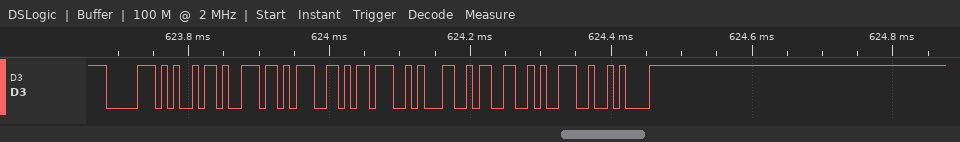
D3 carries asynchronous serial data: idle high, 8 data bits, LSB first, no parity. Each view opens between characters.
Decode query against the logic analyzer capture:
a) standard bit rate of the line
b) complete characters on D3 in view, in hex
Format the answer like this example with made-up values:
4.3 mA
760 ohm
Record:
115200 baud
70, 69, 6E, 67, 3B, 31, 33, 39, 0A
